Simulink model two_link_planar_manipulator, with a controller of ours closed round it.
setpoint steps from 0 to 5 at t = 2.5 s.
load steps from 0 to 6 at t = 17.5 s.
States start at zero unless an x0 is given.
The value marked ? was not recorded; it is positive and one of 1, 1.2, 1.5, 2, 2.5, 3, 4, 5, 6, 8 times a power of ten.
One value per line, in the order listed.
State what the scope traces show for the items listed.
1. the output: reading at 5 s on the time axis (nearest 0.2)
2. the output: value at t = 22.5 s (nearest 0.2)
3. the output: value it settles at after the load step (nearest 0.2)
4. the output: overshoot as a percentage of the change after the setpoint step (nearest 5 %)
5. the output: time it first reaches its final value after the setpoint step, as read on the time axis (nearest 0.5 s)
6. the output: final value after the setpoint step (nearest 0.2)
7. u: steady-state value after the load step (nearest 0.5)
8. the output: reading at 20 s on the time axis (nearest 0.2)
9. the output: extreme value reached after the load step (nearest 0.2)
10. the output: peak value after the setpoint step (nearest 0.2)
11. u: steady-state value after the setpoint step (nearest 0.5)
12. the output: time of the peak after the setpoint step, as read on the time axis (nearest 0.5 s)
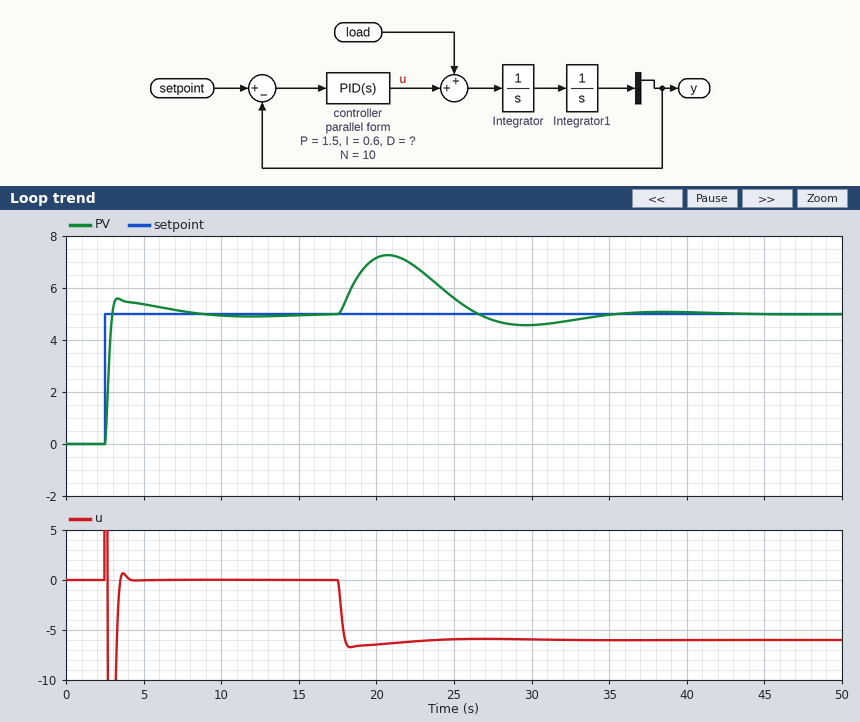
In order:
5.4
6.8
5.0
10 %
3.0 s
5.0
-6.0
7.2
7.2
5.6
0.0
3.5 s
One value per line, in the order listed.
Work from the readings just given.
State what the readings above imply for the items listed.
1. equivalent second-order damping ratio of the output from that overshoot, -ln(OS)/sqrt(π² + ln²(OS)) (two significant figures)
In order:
0.59
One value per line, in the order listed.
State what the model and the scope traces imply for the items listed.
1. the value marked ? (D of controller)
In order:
4
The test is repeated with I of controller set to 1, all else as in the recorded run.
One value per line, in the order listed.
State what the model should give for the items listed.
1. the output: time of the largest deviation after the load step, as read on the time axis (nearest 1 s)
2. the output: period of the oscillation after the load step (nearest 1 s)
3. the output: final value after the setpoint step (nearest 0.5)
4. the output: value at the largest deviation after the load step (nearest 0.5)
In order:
20 s
13 s
5.0
7.0
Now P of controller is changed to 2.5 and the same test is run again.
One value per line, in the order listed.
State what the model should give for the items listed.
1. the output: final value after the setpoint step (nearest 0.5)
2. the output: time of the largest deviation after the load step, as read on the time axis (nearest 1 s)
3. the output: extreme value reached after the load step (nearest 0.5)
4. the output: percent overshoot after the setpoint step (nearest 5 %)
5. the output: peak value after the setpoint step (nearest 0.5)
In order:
5.0
20 s
6.5
15 %
6.0
